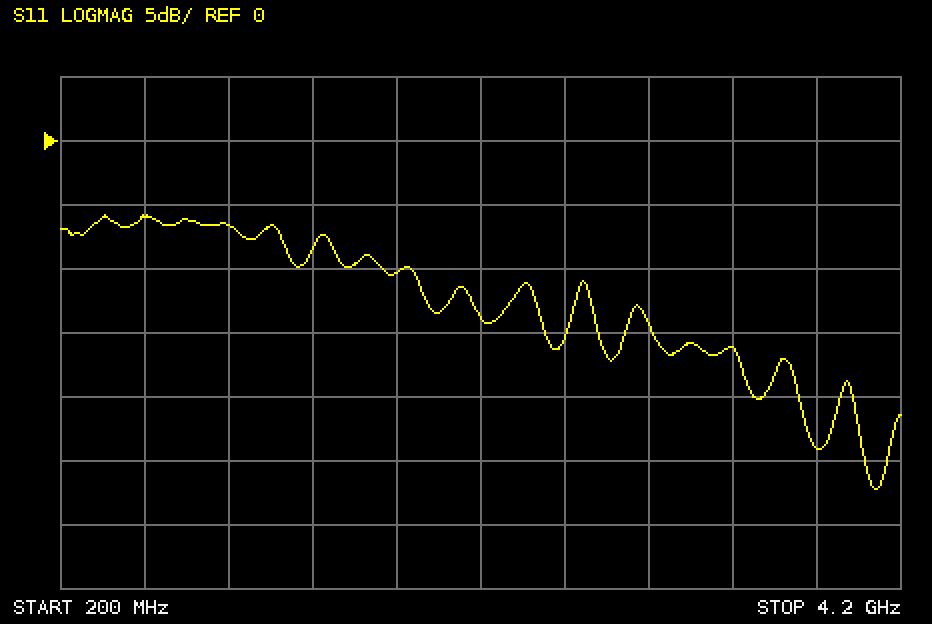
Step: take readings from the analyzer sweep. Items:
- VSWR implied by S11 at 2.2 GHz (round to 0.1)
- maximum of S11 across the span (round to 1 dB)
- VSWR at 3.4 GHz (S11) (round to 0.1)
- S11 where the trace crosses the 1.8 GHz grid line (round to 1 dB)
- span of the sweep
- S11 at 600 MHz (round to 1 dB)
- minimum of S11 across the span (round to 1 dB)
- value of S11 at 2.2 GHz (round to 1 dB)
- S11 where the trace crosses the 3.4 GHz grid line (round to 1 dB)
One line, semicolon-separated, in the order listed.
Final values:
1.5; -6 dB; 1.4; -10 dB; 4 GHz; -6 dB; -27 dB; -14 dB; -16 dB
